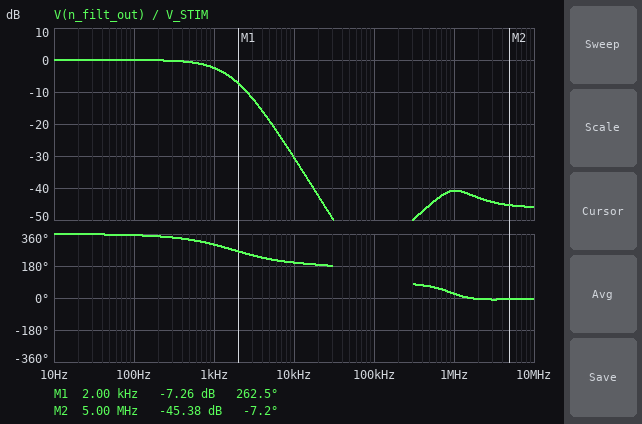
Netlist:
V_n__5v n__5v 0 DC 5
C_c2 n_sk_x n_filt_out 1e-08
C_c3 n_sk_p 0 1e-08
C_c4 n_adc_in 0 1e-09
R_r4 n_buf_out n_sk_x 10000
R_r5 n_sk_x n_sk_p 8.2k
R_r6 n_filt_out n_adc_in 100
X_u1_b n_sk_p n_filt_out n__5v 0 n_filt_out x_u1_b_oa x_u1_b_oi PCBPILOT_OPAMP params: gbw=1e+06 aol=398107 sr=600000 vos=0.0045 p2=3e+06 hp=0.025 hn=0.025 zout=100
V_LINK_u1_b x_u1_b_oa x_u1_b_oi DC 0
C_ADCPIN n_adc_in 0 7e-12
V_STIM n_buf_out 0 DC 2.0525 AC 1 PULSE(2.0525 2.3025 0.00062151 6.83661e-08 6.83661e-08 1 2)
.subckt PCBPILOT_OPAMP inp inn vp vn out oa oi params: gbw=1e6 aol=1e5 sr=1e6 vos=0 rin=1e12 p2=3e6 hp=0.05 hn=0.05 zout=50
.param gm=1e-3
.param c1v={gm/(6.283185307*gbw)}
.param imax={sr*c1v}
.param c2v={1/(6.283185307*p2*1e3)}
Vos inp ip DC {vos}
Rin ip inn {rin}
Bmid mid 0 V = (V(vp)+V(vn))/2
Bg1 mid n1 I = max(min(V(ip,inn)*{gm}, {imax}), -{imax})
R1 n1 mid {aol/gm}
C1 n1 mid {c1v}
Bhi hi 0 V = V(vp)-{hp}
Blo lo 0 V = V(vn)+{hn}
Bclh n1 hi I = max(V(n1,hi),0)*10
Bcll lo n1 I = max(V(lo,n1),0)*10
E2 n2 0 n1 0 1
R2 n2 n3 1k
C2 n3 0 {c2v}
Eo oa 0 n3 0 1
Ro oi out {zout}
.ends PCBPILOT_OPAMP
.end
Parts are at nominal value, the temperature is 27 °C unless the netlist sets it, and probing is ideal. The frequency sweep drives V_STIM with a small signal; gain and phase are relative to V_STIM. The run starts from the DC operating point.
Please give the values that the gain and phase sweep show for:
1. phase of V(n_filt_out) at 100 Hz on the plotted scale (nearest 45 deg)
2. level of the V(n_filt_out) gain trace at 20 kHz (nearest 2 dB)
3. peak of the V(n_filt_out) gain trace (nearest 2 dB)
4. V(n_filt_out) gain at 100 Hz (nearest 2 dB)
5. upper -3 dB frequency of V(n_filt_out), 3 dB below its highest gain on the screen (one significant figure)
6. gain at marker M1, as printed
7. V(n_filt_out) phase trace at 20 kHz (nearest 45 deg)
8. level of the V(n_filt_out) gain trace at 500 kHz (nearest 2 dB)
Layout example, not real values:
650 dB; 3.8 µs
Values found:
360 deg; -42 dB; 0 dB; 0 dB; 1 kHz; -7.26 dB; 180 deg; -46 dB
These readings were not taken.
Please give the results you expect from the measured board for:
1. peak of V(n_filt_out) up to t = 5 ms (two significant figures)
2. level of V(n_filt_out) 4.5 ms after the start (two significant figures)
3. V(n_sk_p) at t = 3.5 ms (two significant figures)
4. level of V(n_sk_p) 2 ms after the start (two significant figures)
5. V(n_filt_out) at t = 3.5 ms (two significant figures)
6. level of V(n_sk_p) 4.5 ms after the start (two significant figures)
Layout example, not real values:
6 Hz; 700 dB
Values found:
2.3 V; 2.3 V; 2.3 V; 2.3 V; 2.3 V; 2.3 V
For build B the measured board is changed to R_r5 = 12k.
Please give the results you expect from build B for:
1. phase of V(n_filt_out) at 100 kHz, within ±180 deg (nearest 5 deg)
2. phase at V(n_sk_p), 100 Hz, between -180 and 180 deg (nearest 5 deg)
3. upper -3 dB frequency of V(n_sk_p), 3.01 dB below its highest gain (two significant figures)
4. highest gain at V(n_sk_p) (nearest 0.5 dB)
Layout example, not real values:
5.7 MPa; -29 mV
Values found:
100 deg; -10 deg; 930 Hz; 0 dB
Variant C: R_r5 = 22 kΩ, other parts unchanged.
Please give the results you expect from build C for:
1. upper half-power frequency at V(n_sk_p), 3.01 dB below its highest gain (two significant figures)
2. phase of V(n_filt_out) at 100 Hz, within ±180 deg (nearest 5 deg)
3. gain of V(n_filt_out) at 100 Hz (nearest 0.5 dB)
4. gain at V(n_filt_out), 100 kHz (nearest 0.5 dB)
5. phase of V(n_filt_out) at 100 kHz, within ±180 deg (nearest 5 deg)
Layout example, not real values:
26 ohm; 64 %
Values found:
620 Hz; -10 deg; 0 dB; -60.0 dB; 95 deg
